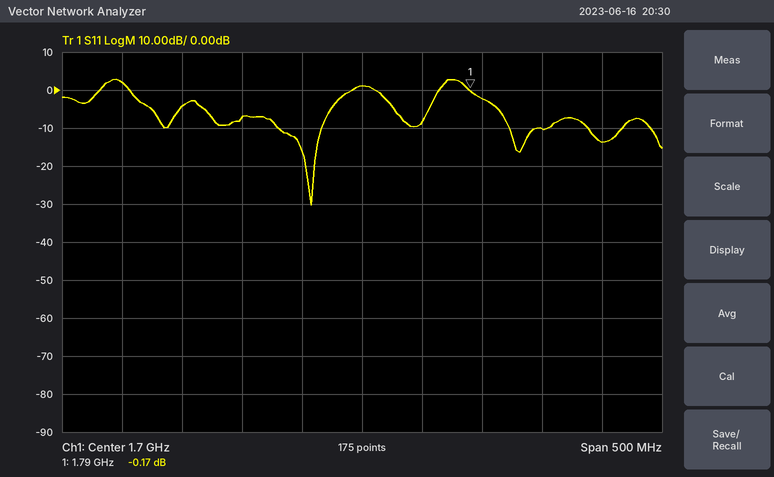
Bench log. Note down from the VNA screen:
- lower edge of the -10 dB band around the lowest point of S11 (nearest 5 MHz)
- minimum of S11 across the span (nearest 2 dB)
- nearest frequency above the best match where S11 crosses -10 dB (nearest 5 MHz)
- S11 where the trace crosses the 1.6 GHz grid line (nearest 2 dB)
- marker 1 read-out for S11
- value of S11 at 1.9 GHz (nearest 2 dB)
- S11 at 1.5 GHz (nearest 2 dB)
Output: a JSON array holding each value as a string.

["1.630 GHz", "-30 dB", "1.665 GHz", "-8 dB", "-0.17 dB", "-14 dB", "2 dB"]
